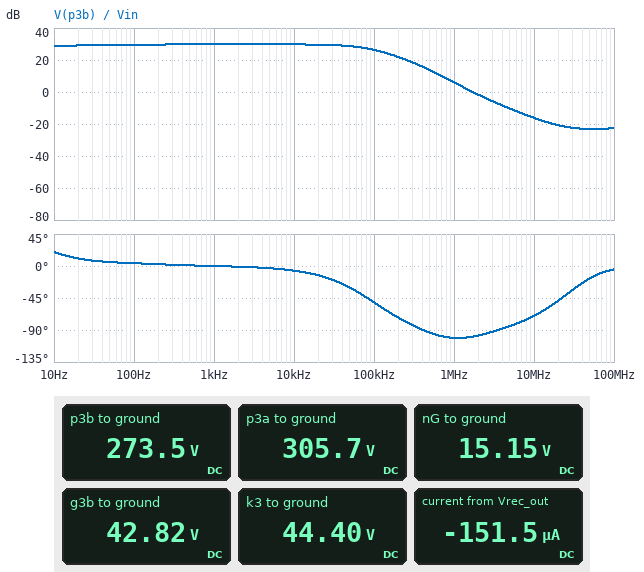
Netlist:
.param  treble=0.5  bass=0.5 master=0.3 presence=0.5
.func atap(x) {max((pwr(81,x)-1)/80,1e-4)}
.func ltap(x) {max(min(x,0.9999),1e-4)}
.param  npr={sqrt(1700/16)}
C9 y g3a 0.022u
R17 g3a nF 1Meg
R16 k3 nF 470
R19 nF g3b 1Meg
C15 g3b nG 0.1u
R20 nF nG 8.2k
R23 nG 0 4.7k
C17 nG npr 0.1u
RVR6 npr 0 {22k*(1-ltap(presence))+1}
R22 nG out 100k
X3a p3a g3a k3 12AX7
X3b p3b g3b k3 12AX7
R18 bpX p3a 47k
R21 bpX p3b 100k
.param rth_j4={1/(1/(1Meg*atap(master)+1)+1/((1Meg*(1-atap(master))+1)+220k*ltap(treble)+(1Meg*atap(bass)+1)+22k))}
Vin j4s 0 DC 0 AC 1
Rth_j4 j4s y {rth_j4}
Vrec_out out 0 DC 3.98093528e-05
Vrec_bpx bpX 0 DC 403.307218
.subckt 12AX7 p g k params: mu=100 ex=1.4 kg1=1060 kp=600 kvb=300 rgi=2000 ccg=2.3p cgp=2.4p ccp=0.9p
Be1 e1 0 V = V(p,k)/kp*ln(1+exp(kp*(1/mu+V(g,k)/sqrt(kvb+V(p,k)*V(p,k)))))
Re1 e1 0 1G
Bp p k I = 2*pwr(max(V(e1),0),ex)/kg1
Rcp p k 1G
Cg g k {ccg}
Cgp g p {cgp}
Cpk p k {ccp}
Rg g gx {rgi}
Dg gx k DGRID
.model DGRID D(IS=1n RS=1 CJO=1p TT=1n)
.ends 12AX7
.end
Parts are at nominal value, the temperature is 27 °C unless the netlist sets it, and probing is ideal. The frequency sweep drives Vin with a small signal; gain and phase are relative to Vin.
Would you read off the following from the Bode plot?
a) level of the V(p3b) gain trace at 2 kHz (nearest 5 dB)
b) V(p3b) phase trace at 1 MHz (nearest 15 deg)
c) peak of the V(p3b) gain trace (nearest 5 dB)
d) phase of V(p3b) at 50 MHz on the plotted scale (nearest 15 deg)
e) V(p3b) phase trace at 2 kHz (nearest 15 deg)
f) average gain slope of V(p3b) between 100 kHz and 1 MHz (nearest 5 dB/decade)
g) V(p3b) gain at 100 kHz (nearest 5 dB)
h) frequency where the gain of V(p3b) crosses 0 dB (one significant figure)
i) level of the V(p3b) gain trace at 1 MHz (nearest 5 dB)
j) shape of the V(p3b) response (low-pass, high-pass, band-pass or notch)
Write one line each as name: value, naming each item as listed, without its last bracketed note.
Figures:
level of the V(p3b) gain trace at 2 kHz: 30 dB
V(p3b) phase trace at 1 MHz: -105 deg
peak of the V(p3b) gain trace: 30 dB
phase of V(p3b) at 50 MHz on the plotted scale: -15 deg
V(p3b) phase trace at 2 kHz: 0 deg
average gain slope of V(p3b) between 100 kHz and 1 MHz: -20 dB/decade
V(p3b) gain at 100 kHz: 25 dB
frequency where the gain of V(p3b) crosses 0 dB: 2 MHz
level of the V(p3b) gain trace at 1 MHz: 5 dB
shape of the V(p3b) response: low-pass
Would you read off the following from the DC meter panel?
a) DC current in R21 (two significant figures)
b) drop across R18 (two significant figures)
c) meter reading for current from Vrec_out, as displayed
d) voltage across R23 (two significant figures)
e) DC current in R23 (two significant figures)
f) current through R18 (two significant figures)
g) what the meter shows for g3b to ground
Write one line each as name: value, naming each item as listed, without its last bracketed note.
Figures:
DC current in R21: 1.3 mA
drop across R18: 98 V
meter reading for current from Vrec_out, as displayed: -151.5 µA
voltage across R23: 15 V
DC current in R23: 3.2 mA
current through R18: 2.1 mA
what the meter shows for g3b to ground: 42.82 V
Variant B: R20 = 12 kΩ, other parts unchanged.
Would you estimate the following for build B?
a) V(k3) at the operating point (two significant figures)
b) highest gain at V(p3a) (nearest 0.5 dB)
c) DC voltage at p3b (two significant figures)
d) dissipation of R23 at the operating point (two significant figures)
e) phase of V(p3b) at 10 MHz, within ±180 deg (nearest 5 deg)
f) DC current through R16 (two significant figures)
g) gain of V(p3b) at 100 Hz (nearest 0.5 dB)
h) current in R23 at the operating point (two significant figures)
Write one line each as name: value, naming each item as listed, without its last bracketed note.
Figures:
V(k3) at the operating point: 55 V
highest gain at V(p3a): 25.0 dB
DC voltage at p3b: 280 V
dissipation of R23 at the operating point: 46 mW
phase of V(p3b) at 10 MHz, within ±180 deg: -70 deg
DC current through R16: 3.3 mA
gain of V(p3b) at 100 Hz: 30.0 dB
current in R23 at the operating point: 3.1 mA
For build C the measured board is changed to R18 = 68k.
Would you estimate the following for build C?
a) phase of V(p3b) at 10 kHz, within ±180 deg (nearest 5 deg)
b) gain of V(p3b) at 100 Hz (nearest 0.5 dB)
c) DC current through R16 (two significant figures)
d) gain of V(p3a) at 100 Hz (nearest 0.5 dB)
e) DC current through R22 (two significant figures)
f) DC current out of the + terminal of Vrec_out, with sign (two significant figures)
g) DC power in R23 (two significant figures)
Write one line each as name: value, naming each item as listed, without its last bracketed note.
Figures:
phase of V(p3b) at 10 kHz, within ±180 deg: -10 deg
gain of V(p3b) at 100 Hz: 29.0 dB
DC current through R16: 3.2 mA
gain of V(p3a) at 100 Hz: 27.0 dB
DC current through R22: 140 µA
DC current out of the + terminal of Vrec_out, with sign: -140 µA
DC power in R23: 43 mW
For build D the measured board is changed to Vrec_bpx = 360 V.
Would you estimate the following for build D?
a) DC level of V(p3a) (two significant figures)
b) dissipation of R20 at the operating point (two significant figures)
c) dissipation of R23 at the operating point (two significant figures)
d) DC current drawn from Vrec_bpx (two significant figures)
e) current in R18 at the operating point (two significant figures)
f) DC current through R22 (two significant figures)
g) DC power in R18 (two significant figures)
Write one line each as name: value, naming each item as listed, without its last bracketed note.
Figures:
DC level of V(p3a): 270 V
dissipation of R20 at the operating point: 73 mW
dissipation of R23 at the operating point: 38 mW
DC current drawn from Vrec_bpx: 3.0 mA
current in R18 at the operating point: 1.8 mA
DC current through R22: 130 µA
DC power in R18: 160 mW
